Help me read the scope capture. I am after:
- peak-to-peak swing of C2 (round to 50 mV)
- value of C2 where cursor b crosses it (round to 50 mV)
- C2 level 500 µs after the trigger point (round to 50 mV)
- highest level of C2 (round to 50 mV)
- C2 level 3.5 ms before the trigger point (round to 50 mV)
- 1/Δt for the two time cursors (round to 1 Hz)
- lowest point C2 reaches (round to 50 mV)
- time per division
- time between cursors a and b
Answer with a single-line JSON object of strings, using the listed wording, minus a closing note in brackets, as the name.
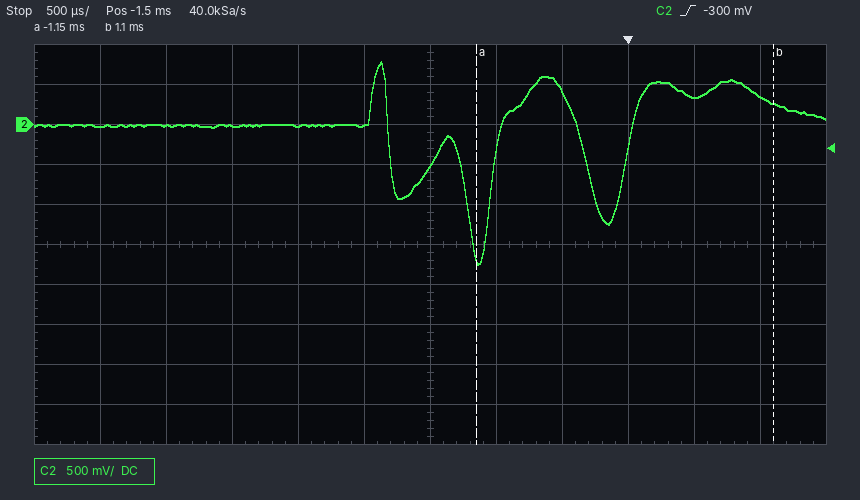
{"peak-to-peak swing of C2": "2.55 V", "value of C2 where cursor b crosses it": "250 mV", "C2 level 500 µs after the trigger point": "350 mV", "highest level of C2": "800 mV", "C2 level 3.5 ms before the trigger point": "0 mV", "1/Δt for the two time cursors": "444 Hz", "lowest point C2 reaches": "-1.75 V", "time per division": "500 µs", "time between cursors a and b": "2.25 ms"}
